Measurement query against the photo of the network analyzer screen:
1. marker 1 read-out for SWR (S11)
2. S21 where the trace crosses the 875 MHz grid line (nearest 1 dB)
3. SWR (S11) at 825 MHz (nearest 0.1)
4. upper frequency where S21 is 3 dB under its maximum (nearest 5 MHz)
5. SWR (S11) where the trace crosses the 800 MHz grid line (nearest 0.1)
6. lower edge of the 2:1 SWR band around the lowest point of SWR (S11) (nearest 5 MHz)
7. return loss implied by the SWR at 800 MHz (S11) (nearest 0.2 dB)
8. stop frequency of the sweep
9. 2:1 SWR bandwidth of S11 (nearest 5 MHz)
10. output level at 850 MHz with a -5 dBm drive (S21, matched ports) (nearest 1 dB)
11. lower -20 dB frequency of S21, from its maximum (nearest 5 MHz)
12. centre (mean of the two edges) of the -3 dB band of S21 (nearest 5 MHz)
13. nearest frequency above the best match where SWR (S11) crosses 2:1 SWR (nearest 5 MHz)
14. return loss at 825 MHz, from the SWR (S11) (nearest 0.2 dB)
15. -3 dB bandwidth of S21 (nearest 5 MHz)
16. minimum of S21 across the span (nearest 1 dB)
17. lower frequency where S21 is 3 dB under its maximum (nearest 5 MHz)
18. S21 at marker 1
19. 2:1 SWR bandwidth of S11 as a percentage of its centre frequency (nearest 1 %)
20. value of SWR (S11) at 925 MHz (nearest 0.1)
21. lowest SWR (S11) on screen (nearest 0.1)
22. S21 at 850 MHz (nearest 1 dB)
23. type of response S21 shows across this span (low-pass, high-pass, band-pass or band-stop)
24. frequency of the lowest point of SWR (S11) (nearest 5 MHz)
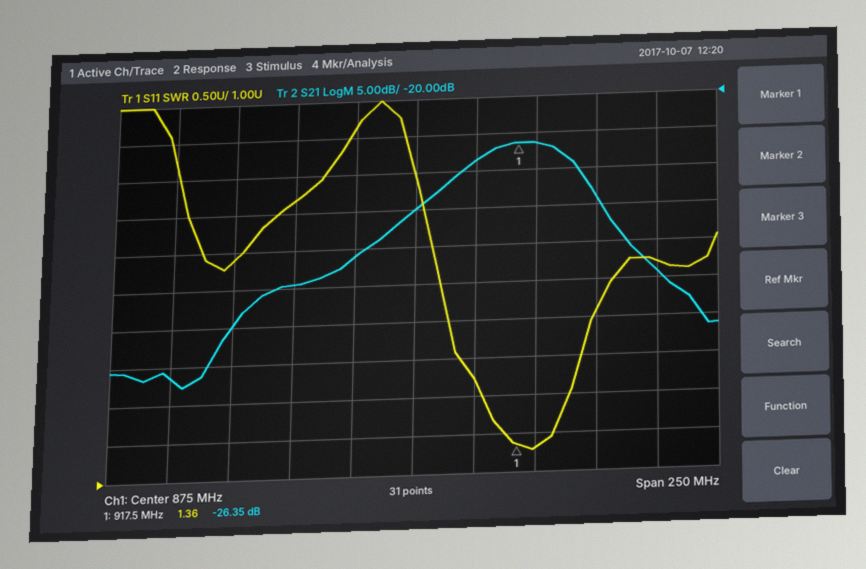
1.36
-35 dB
4.7
940 MHz
3.9
905 MHz
4.6 dB
1 GHz
35 MHz
-46 dBm
810 MHz
920 MHz
940 MHz
3.8 dB
45 MHz
-58 dB
895 MHz
-26.35 dB
4 %
1.3
1.3
-41 dB
band-pass
925 MHz
